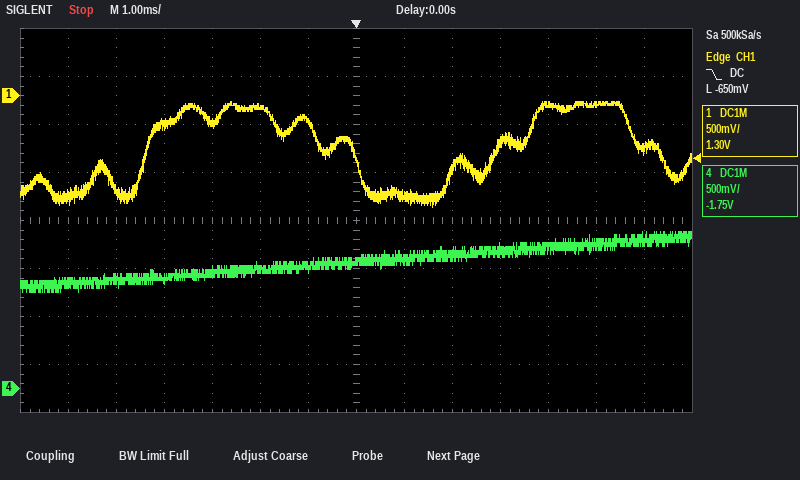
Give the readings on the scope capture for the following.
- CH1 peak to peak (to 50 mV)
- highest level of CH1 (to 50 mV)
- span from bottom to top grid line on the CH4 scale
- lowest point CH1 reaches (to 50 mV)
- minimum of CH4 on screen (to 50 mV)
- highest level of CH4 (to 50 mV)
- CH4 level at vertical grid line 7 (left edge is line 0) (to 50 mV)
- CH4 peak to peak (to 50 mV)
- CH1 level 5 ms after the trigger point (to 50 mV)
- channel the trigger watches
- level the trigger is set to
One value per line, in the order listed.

1.10 V
-50 mV
4 V
-1.15 V
1.00 V
1.65 V
1.30 V
650 mV
-100 mV
CH1
-650 mV
